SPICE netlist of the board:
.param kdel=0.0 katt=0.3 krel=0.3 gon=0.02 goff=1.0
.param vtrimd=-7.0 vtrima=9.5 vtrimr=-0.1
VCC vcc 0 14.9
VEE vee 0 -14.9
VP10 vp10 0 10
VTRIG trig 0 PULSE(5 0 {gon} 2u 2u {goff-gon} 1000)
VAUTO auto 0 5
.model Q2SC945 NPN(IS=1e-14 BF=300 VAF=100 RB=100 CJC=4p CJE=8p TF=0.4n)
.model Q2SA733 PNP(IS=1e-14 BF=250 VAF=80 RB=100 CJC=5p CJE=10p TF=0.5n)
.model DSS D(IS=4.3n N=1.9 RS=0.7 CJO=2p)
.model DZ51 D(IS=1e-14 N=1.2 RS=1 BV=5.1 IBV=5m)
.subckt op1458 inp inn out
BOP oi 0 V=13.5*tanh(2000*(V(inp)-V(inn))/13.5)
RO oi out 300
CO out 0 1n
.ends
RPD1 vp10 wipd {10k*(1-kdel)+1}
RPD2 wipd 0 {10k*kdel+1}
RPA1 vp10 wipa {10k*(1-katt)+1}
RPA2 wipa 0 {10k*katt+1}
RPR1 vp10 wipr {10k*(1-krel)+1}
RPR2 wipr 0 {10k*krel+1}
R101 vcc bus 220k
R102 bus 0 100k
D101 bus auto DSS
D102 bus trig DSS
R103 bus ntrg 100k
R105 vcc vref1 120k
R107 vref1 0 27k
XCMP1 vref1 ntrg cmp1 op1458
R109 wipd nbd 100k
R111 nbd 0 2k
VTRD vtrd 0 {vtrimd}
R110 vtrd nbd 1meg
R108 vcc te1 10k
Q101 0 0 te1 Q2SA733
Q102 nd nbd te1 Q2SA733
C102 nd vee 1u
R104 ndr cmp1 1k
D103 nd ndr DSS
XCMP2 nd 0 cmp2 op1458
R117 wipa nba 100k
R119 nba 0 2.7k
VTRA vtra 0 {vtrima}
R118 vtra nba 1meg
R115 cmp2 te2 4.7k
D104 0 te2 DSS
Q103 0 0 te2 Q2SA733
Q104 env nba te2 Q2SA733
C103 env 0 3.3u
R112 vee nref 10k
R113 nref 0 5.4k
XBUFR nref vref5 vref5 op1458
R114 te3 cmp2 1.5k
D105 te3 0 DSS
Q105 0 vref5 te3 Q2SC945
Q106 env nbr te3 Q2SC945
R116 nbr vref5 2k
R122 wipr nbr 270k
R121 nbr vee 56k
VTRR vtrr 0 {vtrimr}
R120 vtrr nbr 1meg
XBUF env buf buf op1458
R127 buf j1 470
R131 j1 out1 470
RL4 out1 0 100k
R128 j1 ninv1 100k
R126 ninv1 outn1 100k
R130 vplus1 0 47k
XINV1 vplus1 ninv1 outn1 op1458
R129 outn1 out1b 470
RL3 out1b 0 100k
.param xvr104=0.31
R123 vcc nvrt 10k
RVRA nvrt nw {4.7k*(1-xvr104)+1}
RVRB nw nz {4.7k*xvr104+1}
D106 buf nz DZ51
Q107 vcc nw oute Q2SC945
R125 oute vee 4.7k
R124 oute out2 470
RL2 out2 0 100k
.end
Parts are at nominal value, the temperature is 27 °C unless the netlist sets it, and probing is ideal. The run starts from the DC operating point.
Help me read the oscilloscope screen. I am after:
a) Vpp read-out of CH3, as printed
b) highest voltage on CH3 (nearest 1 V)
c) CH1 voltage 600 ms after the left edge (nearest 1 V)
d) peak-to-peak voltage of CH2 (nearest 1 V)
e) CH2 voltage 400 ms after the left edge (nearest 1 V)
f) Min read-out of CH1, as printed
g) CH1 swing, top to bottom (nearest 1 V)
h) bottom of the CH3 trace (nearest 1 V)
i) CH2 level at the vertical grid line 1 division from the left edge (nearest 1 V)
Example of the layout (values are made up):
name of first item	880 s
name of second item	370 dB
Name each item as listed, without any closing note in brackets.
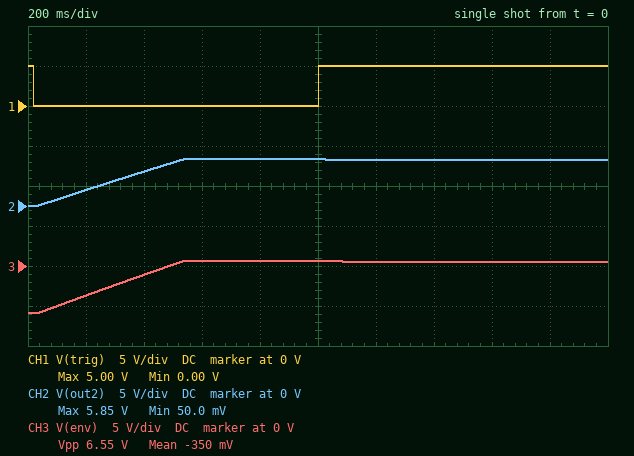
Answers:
Vpp read-out of CH3, as printed	6.55 V
highest voltage on CH3	1 V
CH1 voltage 600 ms after the left edge	0 V
peak-to-peak voltage of CH2	6 V
CH2 voltage 400 ms after the left edge	4 V
Min read-out of CH1, as printed	0.00 V
CH1 swing, top to bottom	5 V
bottom of the CH3 trace	-6 V
CH2 level at the vertical grid line 1 division from the left edge	2 V
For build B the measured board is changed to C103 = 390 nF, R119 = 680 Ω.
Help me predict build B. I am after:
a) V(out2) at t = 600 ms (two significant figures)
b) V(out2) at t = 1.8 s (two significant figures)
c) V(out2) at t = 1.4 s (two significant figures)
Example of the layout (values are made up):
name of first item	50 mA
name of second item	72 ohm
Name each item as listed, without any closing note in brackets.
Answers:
V(out2) at t = 600 ms	5.9 V
V(out2) at t = 1.8 s	5.4 V
V(out2) at t = 1.4 s	5.5 V
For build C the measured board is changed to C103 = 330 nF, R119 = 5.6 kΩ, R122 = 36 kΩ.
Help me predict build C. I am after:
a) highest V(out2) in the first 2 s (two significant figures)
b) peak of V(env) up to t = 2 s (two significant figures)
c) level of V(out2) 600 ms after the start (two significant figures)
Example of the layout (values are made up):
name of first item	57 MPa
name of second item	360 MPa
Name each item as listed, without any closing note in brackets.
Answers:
highest V(out2) in the first 2 s	2.5 V
peak of V(env) up to t = 2 s	-3.1 V
level of V(out2) 600 ms after the start	1.6 V
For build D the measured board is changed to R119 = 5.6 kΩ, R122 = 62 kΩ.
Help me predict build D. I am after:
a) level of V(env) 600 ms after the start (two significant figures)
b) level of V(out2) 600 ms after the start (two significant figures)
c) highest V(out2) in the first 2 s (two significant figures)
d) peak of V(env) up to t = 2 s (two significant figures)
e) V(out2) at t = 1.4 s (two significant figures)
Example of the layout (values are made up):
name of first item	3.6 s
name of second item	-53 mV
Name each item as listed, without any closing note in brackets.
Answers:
level of V(env) 600 ms after the start	-5.6 V
level of V(out2) 600 ms after the start	280 mV
highest V(out2) in the first 2 s	380 mV
peak of V(env) up to t = 2 s	-5.5 V
V(out2) at t = 1.4 s	29 mV
